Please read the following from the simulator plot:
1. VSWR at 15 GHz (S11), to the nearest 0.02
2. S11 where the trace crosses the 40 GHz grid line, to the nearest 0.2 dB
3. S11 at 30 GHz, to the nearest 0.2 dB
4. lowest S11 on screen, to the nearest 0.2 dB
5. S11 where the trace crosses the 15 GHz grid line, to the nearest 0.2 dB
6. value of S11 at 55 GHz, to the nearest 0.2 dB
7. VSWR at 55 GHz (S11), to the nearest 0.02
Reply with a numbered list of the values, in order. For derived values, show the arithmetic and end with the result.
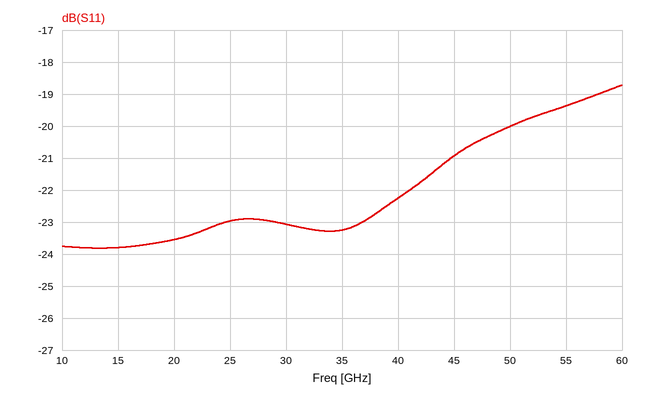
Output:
1. |Γ| = 10^(-23.8/20) = 0.0646; VSWR = (1 + 0.0646)/(1 − 0.0646) ≈ 1.14
2. -22.2 dB
3. -23.0 dB
4. -23.8 dB
5. -23.8 dB
6. -19.4 dB
7. |Γ| = 10^(-19.4/20) = 0.1072; VSWR = (1 + 0.1072)/(1 − 0.1072) ≈ 1.24
